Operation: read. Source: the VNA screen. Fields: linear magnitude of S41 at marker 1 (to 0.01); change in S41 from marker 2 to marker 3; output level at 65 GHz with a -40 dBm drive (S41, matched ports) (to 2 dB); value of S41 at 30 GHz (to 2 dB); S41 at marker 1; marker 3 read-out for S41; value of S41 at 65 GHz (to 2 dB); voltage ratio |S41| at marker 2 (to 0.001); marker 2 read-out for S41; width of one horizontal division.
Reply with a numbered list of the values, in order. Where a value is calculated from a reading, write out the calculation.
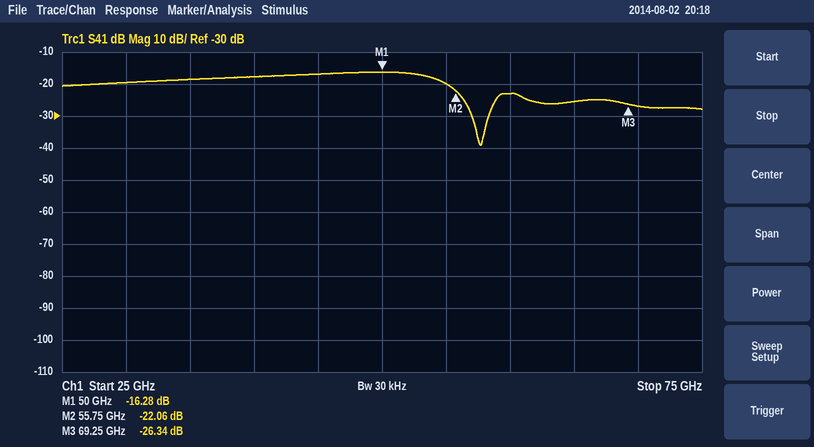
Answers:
1. 10^(-16.28/20) ≈ 0.15
2. -26.34 − (-22.06) = -4.28 dB
3. -40 dBm + (-26 dB) = -66 dBm
4. -20 dB
5. -16.28 dB
6. -26.34 dB
7. -26 dB
8. 10^(-22.06/20) ≈ 0.079
9. -22.06 dB
10. 5 GHz
